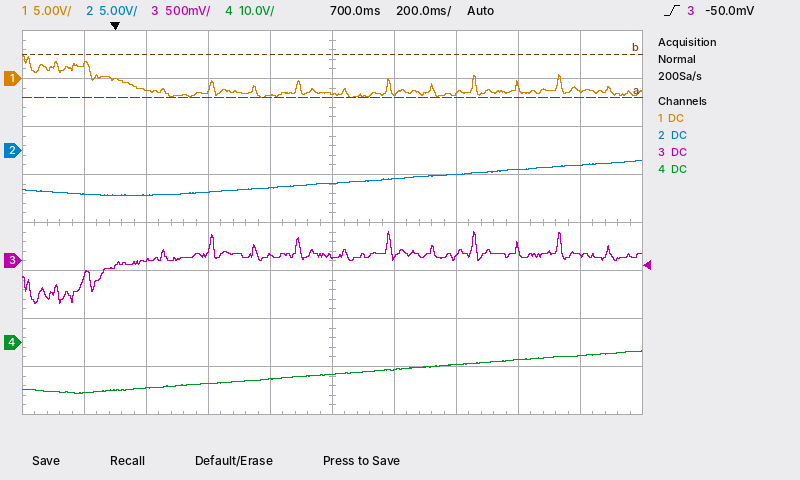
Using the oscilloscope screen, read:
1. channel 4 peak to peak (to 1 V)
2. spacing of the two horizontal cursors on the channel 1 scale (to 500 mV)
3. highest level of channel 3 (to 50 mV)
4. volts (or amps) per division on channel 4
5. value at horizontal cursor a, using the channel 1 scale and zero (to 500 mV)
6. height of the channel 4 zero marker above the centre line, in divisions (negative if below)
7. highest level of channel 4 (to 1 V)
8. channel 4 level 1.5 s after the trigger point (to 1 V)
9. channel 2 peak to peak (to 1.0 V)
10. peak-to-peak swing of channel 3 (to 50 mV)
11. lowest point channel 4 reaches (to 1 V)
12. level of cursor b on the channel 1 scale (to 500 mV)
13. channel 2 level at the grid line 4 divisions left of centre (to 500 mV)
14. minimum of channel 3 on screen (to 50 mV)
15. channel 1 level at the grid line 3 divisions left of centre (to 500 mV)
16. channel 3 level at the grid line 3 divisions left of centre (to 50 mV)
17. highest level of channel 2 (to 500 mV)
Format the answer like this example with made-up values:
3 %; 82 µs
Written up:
9 V; 4.5 V; 300 mV; 10 V; -2.0 V; -2.5 div; -2 V; -3 V; 4.0 V; 750 mV; -11 V; 2.5 V; -4.5 V; -450 mV; -1.0 V; 0 mV; -1.0 V
